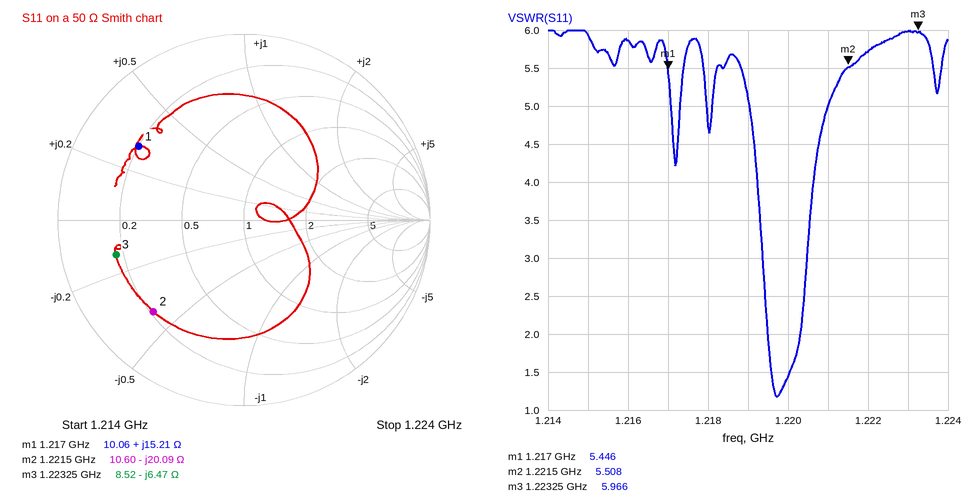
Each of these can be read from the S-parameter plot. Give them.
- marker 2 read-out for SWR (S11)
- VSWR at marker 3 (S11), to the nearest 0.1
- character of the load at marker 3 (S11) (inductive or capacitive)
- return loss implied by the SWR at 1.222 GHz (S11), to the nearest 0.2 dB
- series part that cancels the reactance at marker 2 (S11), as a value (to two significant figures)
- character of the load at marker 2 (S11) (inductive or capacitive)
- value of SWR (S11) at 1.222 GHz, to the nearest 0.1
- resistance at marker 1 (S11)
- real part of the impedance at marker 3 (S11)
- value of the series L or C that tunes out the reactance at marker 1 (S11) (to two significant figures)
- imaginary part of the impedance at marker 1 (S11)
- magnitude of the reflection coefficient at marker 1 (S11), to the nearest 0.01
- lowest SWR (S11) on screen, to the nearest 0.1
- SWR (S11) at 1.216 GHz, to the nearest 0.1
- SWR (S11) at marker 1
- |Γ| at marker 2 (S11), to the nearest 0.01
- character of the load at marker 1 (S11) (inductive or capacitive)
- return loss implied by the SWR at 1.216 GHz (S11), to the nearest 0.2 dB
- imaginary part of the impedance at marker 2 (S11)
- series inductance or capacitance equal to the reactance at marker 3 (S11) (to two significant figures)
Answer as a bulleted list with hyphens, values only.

- 5.508
- 6.0
- capacitive
- 3.0 dB
- 2.6 nH
- capacitive
- 5.7
- 10.06 Ω
- 8.52 Ω
- 8.6 pF
- +15.21 Ω
- 0.69
- 1.2
- 5.9
- 5.446
- 0.69
- inductive
- 3.0 dB
- -20.09 Ω
- 20 pF
